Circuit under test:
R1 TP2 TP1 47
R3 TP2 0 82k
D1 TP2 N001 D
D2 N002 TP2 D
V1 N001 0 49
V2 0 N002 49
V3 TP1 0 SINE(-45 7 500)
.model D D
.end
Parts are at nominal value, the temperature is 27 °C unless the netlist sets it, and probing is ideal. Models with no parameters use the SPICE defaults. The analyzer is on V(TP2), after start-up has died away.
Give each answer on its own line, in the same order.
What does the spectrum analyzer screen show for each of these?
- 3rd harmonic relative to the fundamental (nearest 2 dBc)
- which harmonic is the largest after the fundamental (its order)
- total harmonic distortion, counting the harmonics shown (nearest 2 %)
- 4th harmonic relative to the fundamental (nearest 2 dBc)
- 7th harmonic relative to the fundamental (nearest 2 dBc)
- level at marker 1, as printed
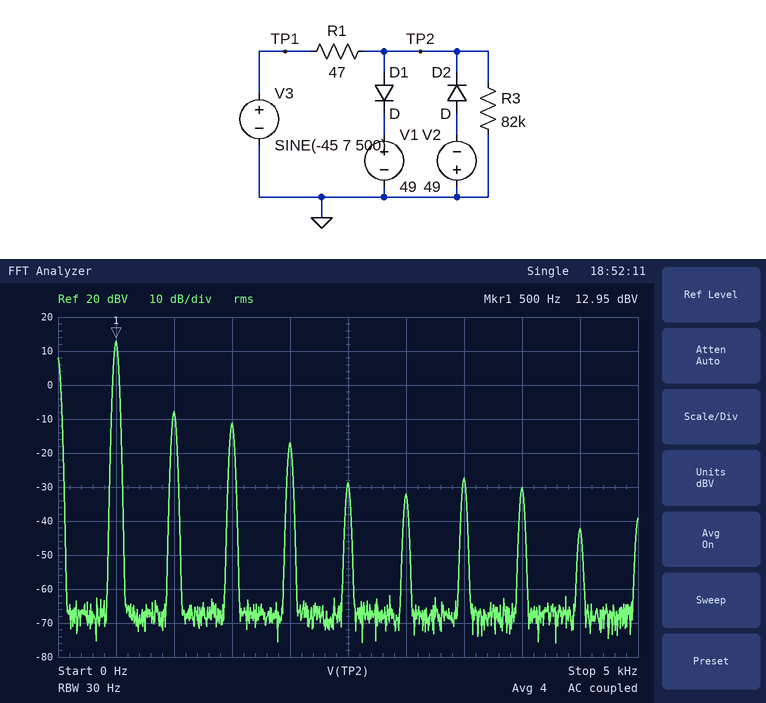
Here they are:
-24 dBc
2
12 %
-30 dBc
-40 dBc
12.95 dBV
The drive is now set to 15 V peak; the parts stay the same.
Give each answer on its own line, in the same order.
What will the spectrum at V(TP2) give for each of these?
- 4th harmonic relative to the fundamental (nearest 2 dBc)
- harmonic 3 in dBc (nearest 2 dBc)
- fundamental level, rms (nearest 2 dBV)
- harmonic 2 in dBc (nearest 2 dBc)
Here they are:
-34 dBc
-22 dBc
18 dBV
-12 dBc
